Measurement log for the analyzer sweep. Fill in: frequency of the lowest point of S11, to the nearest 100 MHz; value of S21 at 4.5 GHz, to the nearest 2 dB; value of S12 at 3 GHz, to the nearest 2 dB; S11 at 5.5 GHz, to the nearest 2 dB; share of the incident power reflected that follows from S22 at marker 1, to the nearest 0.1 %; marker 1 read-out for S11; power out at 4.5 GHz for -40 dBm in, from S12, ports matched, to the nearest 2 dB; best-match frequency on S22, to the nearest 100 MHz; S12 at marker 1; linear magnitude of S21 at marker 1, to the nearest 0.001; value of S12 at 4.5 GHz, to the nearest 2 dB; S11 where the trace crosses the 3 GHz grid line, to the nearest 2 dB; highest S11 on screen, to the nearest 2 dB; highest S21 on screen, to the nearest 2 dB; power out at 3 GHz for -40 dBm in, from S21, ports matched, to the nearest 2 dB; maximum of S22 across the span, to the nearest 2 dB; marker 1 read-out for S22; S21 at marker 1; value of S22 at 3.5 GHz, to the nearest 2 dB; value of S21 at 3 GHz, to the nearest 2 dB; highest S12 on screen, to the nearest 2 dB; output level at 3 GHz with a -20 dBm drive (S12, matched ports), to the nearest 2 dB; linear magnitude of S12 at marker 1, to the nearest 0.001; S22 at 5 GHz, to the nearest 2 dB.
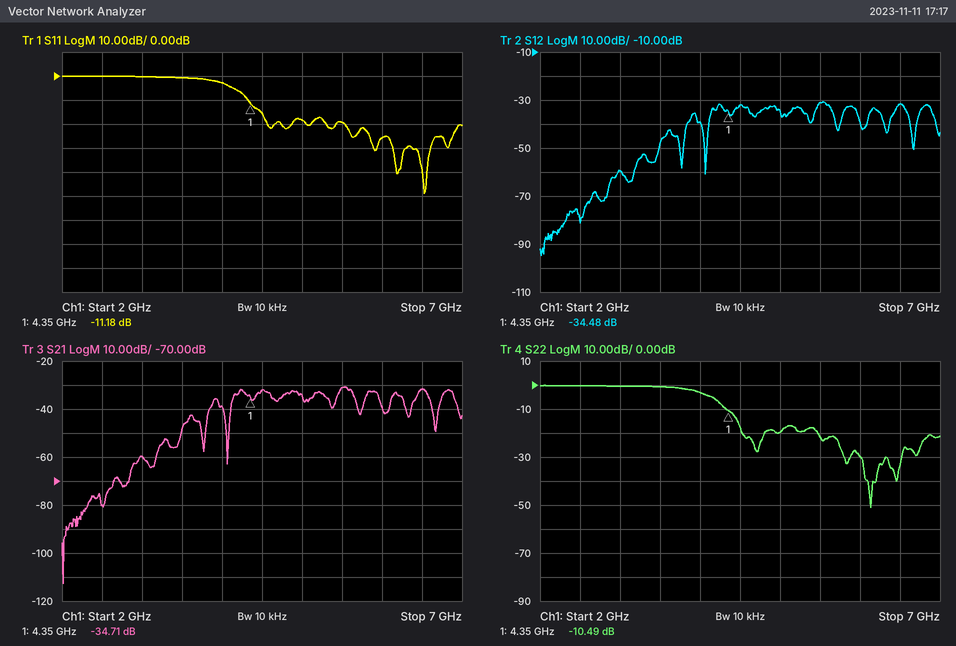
6.5 GHz
-32 dB
-60 dB
-20 dB
8.9 %
-11.18 dB
-72 dBm
6.1 GHz
-34.48 dB
0.018
-32 dB
0 dB
0 dB
-30 dB
-100 dBm
0 dB
-10.49 dB
-34.71 dB
0 dB
-60 dB
-30 dB
-80 dBm
0.019
-20 dB
